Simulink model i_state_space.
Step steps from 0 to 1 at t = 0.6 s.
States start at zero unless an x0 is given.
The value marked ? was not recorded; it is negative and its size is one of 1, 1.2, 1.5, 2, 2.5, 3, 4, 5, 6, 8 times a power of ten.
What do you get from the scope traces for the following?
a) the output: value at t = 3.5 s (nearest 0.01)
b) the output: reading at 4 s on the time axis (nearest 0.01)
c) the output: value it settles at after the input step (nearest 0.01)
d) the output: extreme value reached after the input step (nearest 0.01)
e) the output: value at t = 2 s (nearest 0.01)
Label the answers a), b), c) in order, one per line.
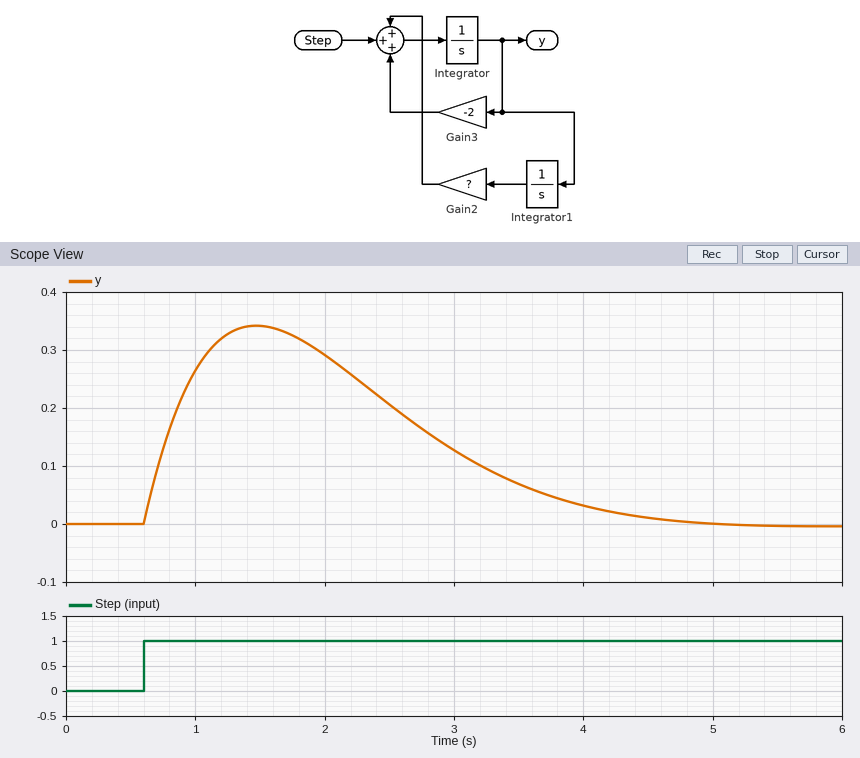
a) 0.07
b) 0.03
c) 0.00
d) 0.34
e) 0.29
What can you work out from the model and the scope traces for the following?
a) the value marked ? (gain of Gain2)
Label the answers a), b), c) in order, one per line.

a) -1.5
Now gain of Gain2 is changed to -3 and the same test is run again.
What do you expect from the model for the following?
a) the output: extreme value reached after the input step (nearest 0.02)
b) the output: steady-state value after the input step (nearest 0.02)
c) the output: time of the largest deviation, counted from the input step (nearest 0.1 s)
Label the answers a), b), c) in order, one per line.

a) 0.30
b) 0.00
c) 0.7 s
